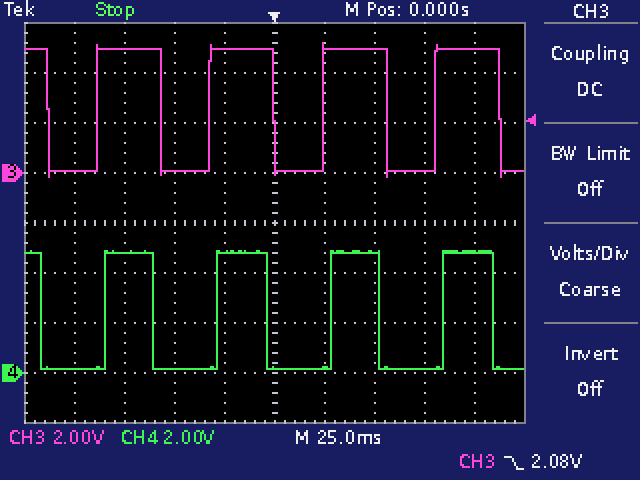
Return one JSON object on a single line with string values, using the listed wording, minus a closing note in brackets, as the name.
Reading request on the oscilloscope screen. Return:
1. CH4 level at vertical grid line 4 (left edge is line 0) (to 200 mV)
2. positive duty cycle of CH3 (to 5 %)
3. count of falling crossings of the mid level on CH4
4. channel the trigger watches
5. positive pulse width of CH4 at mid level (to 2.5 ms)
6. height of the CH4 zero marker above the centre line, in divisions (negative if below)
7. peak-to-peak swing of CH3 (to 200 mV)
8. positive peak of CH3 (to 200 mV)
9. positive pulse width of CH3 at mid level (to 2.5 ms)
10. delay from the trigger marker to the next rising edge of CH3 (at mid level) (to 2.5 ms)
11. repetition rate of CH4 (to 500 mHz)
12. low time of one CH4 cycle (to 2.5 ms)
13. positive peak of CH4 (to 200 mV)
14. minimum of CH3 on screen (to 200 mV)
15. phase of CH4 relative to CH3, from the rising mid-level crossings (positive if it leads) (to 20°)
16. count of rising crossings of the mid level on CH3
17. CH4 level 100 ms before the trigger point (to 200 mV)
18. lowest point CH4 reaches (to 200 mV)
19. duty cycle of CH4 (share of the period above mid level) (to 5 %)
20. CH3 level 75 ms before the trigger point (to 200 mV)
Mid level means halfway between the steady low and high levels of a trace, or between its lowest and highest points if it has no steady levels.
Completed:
{"CH4 level at vertical grid line 4 (left edge is line 0)": "4.8 V", "positive duty cycle of CH3": "55 %", "count of falling crossings of the mid level on CH4": "5", "channel the trigger watches": "CH3", "positive pulse width of CH4 at mid level": "25.0 ms", "height of the CH4 zero marker above the centre line, in divisions": "-3.0 div", "peak-to-peak swing of CH3": "5.4 V", "positive peak of CH3": "5.2 V", "positive pulse width of CH3 at mid level": "32.5 ms", "delay from the trigger marker to the next rising edge of CH3 (at mid level)": "25.0 ms", "repetition rate of CH4": "17.5 Hz", "low time of one CH4 cycle": "32.5 ms", "positive peak of CH4": "4.8 V", "minimum of CH3 on screen": "-200 mV", "phase of CH4 relative to CH3, from the rising mid-level crossings (positive if it leads)": "-20°", "count of rising crossings of the mid level on CH3": "4", "CH4 level 100 ms before the trigger point": "200 mV", "lowest point CH4 reaches": "200 mV", "duty cycle of CH4 (share of the period above mid level)": "45 %", "CH3 level 75 ms before the trigger point": "5.0 V"}
